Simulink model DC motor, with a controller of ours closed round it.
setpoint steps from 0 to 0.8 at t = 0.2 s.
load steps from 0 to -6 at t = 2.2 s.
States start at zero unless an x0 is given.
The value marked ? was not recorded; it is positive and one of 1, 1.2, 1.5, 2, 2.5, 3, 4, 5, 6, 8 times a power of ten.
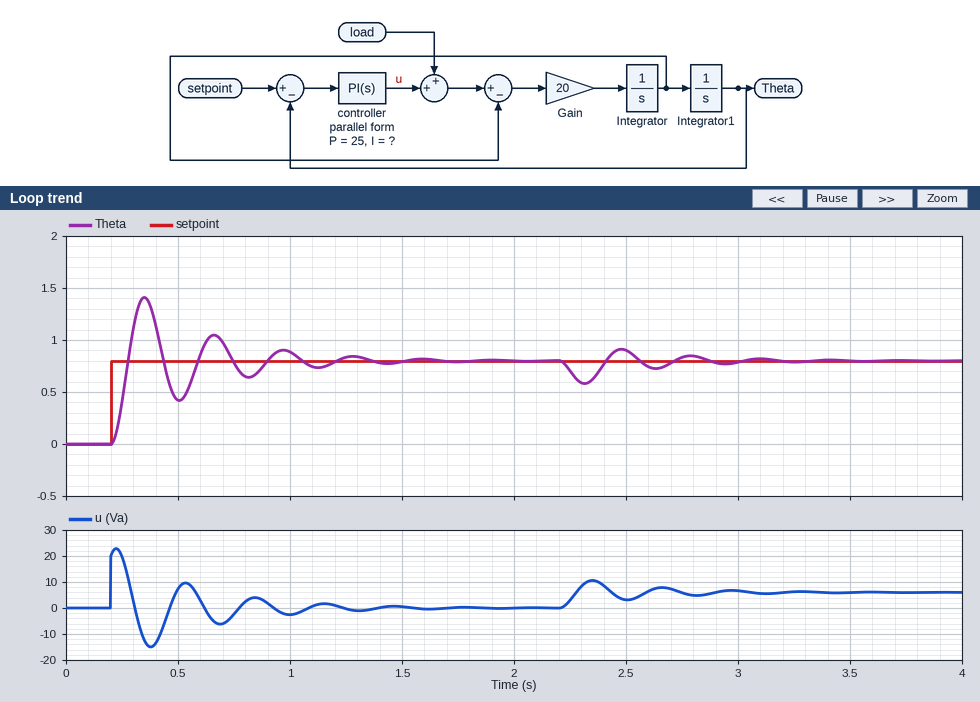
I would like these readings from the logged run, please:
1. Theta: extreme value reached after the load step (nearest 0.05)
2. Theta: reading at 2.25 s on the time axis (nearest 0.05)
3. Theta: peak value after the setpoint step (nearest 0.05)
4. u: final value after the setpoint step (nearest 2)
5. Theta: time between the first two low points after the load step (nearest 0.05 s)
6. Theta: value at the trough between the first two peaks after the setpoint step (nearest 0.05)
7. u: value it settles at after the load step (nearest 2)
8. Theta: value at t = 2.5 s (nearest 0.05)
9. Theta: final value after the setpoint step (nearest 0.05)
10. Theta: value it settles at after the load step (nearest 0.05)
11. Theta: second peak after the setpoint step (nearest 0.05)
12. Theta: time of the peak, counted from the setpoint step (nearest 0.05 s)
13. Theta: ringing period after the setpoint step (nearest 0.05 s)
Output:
0.60
0.70
1.40
0
0.30 s
0.40
6
0.90
0.80
0.80
1.05
0.15 s
0.30 s
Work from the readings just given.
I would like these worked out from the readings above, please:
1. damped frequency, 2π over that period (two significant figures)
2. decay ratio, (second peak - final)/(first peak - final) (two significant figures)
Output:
21 rad/s
0.42
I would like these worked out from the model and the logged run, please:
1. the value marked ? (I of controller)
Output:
300
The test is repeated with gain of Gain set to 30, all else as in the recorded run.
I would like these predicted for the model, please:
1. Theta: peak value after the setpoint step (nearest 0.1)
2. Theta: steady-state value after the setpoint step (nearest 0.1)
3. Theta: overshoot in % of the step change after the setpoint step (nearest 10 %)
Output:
1.3
0.8
60 %
